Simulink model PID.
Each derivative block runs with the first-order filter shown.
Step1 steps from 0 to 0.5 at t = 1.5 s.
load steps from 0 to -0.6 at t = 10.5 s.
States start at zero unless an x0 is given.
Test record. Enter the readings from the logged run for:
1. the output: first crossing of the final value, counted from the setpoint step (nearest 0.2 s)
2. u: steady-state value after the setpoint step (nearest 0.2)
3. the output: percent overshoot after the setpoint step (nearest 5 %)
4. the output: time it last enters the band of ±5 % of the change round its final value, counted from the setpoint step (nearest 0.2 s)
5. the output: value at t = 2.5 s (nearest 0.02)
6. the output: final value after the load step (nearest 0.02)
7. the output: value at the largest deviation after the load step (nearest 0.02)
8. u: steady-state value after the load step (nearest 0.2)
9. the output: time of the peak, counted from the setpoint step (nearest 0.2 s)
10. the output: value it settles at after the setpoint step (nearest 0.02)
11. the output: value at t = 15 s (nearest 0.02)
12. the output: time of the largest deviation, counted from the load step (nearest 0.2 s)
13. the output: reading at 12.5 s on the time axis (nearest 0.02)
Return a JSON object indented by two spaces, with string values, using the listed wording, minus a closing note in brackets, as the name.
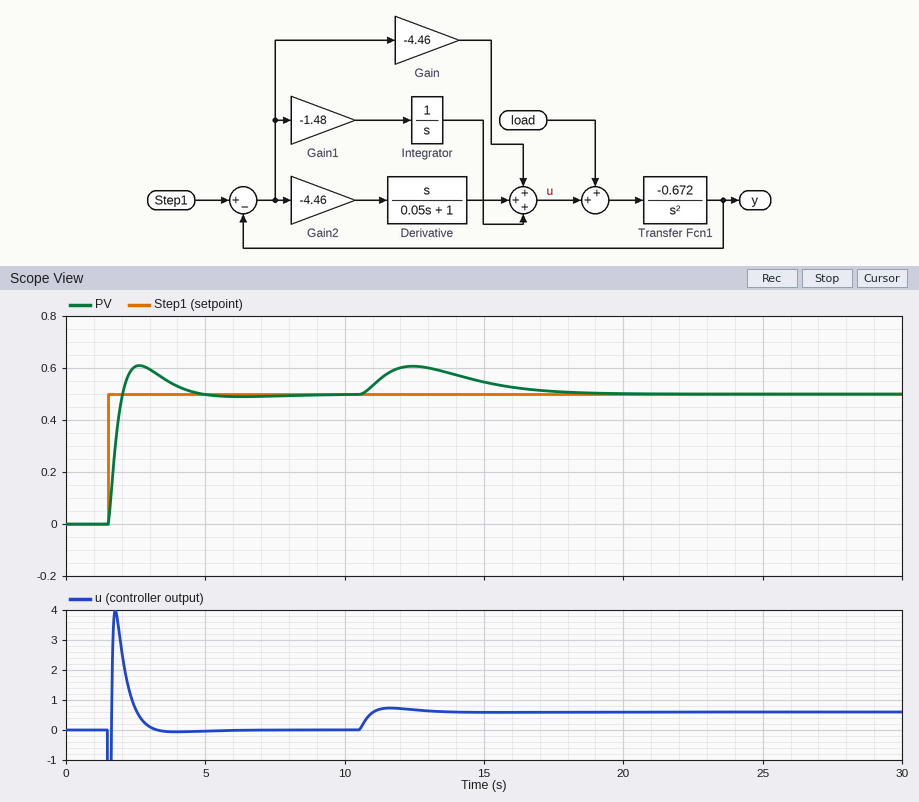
{
  "the output: first crossing of the final value, counted from the setpoint step": "0.6 s",
  "u: steady-state value after the setpoint step": "0.0",
  "the output: percent overshoot after the setpoint step": "20 %",
  "the output: time it last enters the band of ±5 % of the change round its final value, counted from the setpoint step": "2.6 s",
  "the output: value at t = 2.5 s": "0.60",
  "the output: final value after the load step": "0.50",
  "the output: value at the largest deviation after the load step": "0.60",
  "u: steady-state value after the load step": "0.6",
  "the output: time of the peak, counted from the setpoint step": "1.2 s",
  "the output: value it settles at after the setpoint step": "0.50",
  "the output: value at t = 15 s": "0.54",
  "the output: time of the largest deviation, counted from the load step": "2.0 s",
  "the output: reading at 12.5 s on the time axis": "0.60"
}
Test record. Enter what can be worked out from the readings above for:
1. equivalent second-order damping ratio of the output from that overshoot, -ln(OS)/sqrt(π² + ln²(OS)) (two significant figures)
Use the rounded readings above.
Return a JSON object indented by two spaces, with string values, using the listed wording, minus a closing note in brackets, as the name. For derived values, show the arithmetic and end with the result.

{
  "equivalent second-order damping ratio of the output from that overshoot, -ln(OS)/sqrt(π² + ln²(OS))": "ln(0.2) = -1.609; 1.609 / sqrt(9.870 + 2.590) = 0.46"
}
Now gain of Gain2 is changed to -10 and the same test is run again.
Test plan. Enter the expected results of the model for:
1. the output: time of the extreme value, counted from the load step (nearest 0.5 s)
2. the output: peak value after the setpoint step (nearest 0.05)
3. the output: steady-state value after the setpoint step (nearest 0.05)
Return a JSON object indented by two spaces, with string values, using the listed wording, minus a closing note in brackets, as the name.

{
  "the output: time of the extreme value, counted from the load step": "3.0 s",
  "the output: peak value after the setpoint step": "0.55",
  "the output: steady-state value after the setpoint step": "0.50"
}
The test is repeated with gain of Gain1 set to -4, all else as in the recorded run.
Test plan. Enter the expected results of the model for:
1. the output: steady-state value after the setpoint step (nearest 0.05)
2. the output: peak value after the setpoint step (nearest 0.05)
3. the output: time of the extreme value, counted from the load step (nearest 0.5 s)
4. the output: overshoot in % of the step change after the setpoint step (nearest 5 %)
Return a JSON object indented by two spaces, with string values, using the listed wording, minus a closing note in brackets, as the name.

{
  "the output: steady-state value after the setpoint step": "0.50",
  "the output: peak value after the setpoint step": "0.65",
  "the output: time of the extreme value, counted from the load step": "1.5 s",
  "the output: overshoot in % of the step change after the setpoint step": "30 %"
}
